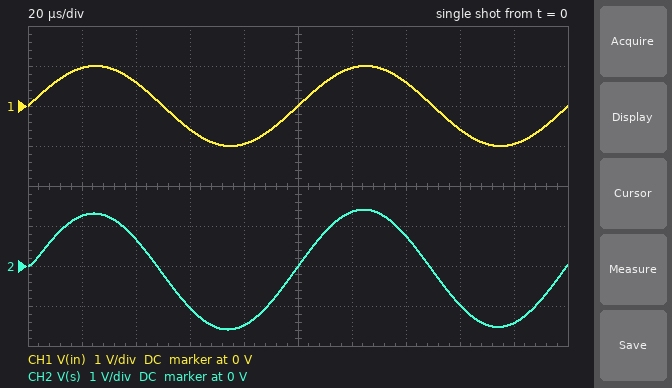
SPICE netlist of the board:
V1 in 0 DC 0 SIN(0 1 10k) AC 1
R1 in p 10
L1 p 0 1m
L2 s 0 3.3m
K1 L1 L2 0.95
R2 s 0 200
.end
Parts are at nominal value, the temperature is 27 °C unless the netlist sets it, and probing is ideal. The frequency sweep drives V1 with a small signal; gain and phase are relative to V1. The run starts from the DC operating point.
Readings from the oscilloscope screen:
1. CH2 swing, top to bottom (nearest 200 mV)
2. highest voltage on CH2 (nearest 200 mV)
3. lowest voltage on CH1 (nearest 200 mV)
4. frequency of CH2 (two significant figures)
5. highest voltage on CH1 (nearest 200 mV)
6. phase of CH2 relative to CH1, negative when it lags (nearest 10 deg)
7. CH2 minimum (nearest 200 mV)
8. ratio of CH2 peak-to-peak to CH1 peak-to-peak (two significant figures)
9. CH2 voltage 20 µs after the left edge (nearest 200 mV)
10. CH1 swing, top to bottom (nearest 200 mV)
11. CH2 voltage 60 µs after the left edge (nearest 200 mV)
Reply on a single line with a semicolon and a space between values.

3.0 V; 1.4 V; -1.0 V; 10 kHz; 1.0 V; 0 deg; -1.6 V; 1.5; 1.2 V; 2.0 V; -1.0 V
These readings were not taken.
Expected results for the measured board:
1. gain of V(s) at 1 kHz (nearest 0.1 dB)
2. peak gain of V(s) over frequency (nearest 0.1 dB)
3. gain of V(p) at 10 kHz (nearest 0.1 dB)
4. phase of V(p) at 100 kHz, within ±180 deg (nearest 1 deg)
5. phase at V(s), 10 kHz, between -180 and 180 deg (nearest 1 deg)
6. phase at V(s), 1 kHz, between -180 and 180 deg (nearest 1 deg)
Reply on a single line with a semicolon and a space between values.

-1.1 dB; 3.4 dB; -1.3 dB; 5 deg; 3 deg; 54 deg
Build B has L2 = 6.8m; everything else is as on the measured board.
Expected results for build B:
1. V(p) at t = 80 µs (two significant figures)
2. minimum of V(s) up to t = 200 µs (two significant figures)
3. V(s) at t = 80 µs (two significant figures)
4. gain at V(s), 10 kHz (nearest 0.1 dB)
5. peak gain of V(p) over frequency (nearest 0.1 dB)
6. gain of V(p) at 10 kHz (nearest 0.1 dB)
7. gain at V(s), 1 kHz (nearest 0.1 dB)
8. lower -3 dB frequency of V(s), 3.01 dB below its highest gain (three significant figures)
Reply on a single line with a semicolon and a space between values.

-720 mV; -2.0 V; -1.9 V; 5.3 dB; 0 dB; -2.4 dB; 1.6 dB; 1.17 kHz
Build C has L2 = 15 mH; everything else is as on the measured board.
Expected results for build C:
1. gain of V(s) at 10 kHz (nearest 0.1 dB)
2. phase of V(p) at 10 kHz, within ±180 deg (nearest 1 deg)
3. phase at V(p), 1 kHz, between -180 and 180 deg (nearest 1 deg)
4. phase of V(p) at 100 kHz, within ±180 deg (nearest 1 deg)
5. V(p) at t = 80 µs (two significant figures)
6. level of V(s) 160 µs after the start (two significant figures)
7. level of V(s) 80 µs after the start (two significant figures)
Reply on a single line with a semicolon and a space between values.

6.3 dB; 15 deg; 44 deg; 9 deg; -550 mV; -1.0 V; -2.2 V
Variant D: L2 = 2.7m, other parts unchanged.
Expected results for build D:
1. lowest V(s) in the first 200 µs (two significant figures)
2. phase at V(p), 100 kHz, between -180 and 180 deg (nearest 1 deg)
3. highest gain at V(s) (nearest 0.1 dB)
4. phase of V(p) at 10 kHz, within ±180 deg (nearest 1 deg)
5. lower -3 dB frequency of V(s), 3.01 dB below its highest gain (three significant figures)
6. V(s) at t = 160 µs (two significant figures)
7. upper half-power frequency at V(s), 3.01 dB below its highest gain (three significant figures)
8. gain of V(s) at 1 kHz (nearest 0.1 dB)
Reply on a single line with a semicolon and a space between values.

-1.5 V; 4 deg; 2.8 dB; 9 deg; 1.39 kHz; -930 mV; 139 kHz; -1.9 dB
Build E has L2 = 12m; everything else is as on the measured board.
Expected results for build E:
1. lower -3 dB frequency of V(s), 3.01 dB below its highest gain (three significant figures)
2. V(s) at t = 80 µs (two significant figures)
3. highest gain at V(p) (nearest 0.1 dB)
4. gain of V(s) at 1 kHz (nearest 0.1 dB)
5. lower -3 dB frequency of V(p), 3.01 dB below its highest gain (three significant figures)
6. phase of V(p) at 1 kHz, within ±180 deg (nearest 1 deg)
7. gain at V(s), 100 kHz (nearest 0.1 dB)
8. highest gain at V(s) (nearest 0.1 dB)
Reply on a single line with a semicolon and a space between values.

973 Hz; -2.1 V; 0 dB; 3.4 dB; 18.3 kHz; 46 deg; -1.7 dB; 6.3 dB
